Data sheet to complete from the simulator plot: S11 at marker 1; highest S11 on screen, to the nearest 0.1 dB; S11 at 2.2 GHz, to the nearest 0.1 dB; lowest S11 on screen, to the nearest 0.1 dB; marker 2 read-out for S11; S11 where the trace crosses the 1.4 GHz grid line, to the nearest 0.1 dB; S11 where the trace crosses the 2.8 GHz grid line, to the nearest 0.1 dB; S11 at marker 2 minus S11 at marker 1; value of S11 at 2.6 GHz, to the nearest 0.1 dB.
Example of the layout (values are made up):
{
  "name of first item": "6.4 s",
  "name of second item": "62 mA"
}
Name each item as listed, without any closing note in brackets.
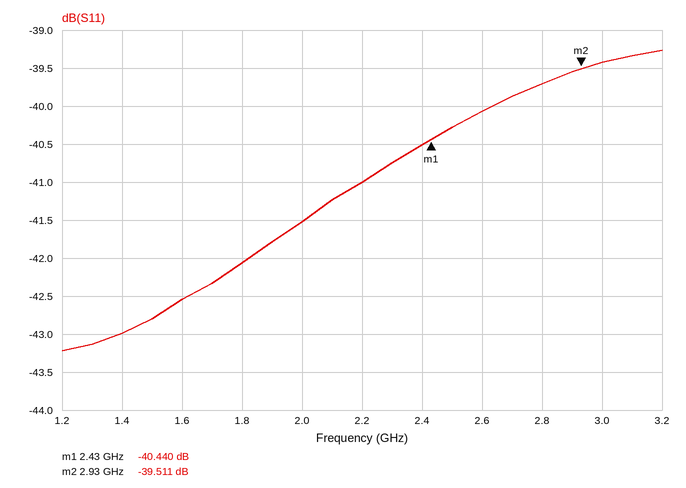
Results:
{
  "S11 at marker 1": "-40.440 dB",
  "highest S11 on screen, to the nearest 0.1 dB": "-39.3 dB",
  "S11 at 2.2 GHz, to the nearest 0.1 dB": "-41.0 dB",
  "lowest S11 on screen, to the nearest 0.1 dB": "-43.2 dB",
  "marker 2 read-out for S11": "-39.511 dB",
  "S11 where the trace crosses the 1.4 GHz grid line, to the nearest 0.1 dB": "-43.0 dB",
  "S11 where the trace crosses the 2.8 GHz grid line, to the nearest 0.1 dB": "-39.7 dB",
  "S11 at marker 2 minus S11 at marker 1": "0.929 dB",
  "value of S11 at 2.6 GHz, to the nearest 0.1 dB": "-40.1 dB"
}
